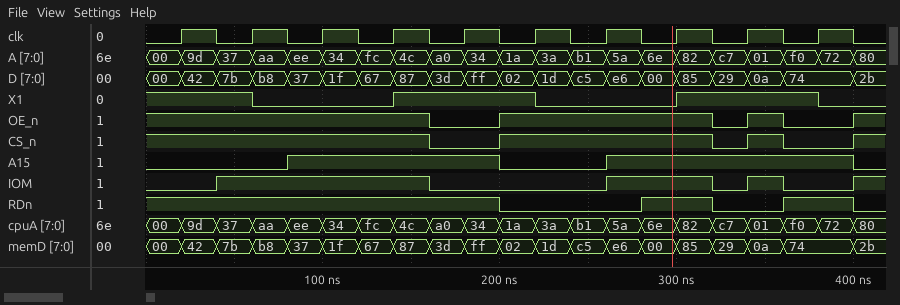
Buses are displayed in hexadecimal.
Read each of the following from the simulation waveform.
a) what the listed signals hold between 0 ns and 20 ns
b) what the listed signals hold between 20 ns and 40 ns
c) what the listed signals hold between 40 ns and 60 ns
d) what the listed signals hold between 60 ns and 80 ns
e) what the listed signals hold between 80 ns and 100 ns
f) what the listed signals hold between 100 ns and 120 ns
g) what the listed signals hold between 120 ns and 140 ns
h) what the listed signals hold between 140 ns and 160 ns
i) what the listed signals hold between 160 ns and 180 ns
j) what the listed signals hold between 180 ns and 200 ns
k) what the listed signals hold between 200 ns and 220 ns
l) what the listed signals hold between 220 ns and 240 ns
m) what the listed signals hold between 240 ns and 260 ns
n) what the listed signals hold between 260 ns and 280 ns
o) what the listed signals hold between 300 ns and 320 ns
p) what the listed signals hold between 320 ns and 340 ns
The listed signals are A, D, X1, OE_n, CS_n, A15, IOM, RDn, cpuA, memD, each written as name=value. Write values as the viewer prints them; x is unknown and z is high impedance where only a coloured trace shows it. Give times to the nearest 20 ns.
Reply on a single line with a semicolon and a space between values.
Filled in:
A=00, D=00, X1=1, OE_n=1, CS_n=1, A15=0, IOM=0, RDn=1, cpuA=00, memD=00; A=9d, D=42, X1=1, OE_n=1, CS_n=1, A15=0, IOM=0, RDn=1, cpuA=9d, memD=42; A=37, D=7b, X1=1, OE_n=1, CS_n=1, A15=0, IOM=1, RDn=1, cpuA=37, memD=7b; A=aa, D=b8, X1=0, OE_n=1, CS_n=1, A15=0, IOM=1, RDn=1, cpuA=aa, memD=b8; A=ee, D=37, X1=0, OE_n=1, CS_n=1, A15=1, IOM=1, RDn=1, cpuA=ee, memD=37; A=34, D=1f, X1=0, OE_n=1, CS_n=1, A15=1, IOM=1, RDn=1, cpuA=34, memD=1f; A=fc, D=67, X1=0, OE_n=1, CS_n=1, A15=1, IOM=1, RDn=1, cpuA=fc, memD=67; A=4c, D=87, X1=1, OE_n=1, CS_n=1, A15=1, IOM=1, RDn=1, cpuA=4c, memD=87; A=a0, D=3d, X1=1, OE_n=0, CS_n=0, A15=1, IOM=0, RDn=1, cpuA=a0, memD=3d; A=34, D=ff, X1=1, OE_n=0, CS_n=0, A15=1, IOM=0, RDn=1, cpuA=34, memD=ff; A=1a, D=02, X1=1, OE_n=1, CS_n=1, A15=0, IOM=0, RDn=0, cpuA=1a, memD=02; A=3a, D=1d, X1=0, OE_n=1, CS_n=1, A15=0, IOM=0, RDn=0, cpuA=3a, memD=1d; A=b1, D=c5, X1=0, OE_n=1, CS_n=1, A15=0, IOM=0, RDn=0, cpuA=b1, memD=c5; A=5a, D=e6, X1=0, OE_n=1, CS_n=1, A15=1, IOM=1, RDn=0, cpuA=5a, memD=e6; A=82, D=85, X1=1, OE_n=1, CS_n=1, A15=1, IOM=1, RDn=1, cpuA=82, memD=85; A=c7, D=29, X1=1, OE_n=0, CS_n=0, A15=1, IOM=0, RDn=0, cpuA=c7, memD=29
